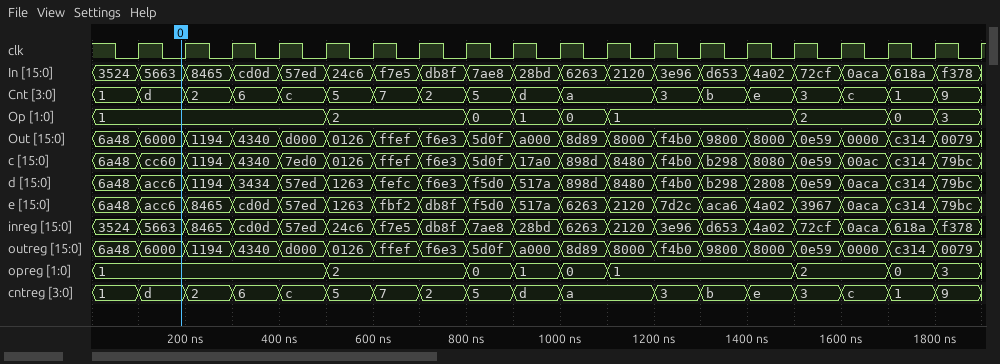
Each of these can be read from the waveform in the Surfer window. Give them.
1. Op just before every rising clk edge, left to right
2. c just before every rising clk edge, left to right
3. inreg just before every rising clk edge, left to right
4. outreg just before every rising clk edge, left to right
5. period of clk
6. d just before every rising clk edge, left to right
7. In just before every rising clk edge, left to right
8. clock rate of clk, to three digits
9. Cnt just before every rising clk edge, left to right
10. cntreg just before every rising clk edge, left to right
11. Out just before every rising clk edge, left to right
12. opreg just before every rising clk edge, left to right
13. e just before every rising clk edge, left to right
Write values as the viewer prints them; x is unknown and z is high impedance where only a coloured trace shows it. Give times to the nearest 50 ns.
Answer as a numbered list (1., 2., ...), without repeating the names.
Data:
1. 1, 1, 1, 1, 1, 2, 2, 2, 0, 1, 0, 1, 1, 1, 1, 2, 2, 0, 3
2. 6a48, cc60, 1194, 4340, 7ed0, 0126, ffef, f6e3, 5d0f, 17a0, 898d, 8480, f4b0, b298, 8080, 0e59, 00ac, c314, 79bc
3. 3524, 5663, 8465, cd0d, 57ed, 24c6, f7e5, db8f, 7ae8, 28bd, 6263, 2120, 3e96, d653, 4a02, 72cf, 0aca, 618a, f378
4. 6a48, 6000, 1194, 4340, d000, 0126, ffef, f6e3, 5d0f, a000, 8d89, 8000, f4b0, 9800, 8000, 0e59, 0000, c314, 0079
5. 100 ns
6. 6a48, acc6, 1194, 3434, 57ed, 1263, fefc, f6e3, f5d0, 517a, 898d, 8480, f4b0, b298, 2808, 0e59, 0aca, c314, 79bc
7. 3524, 5663, 8465, cd0d, 57ed, 24c6, f7e5, db8f, 7ae8, 28bd, 6263, 2120, 3e96, d653, 4a02, 72cf, 0aca, 618a, f378
8. 10.0 MHz
9. 1, d, 2, 6, c, 5, 7, 2, 5, d, a, a, 3, b, e, 3, c, 1, 9
10. 1, d, 2, 6, c, 5, 7, 2, 5, d, a, a, 3, b, e, 3, c, 1, 9
11. 6a48, 6000, 1194, 4340, d000, 0126, ffef, f6e3, 5d0f, a000, 8d89, 8000, f4b0, 9800, 8000, 0e59, 0000, c314, 0079
12. 1, 1, 1, 1, 1, 2, 2, 2, 0, 1, 0, 1, 1, 1, 1, 2, 2, 0, 3
13. 6a48, acc6, 8465, cd0d, 57ed, 1263, fbf2, db8f, f5d0, 517a, 6263, 2120, 7d2c, aca6, 4a02, 3967, 0aca, c314, 79bc
